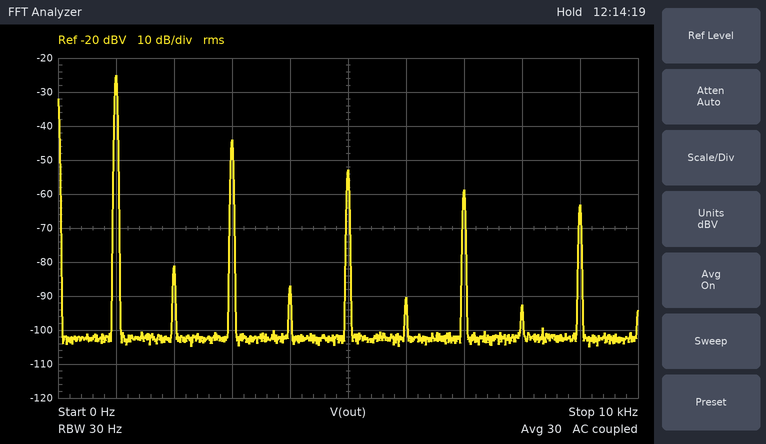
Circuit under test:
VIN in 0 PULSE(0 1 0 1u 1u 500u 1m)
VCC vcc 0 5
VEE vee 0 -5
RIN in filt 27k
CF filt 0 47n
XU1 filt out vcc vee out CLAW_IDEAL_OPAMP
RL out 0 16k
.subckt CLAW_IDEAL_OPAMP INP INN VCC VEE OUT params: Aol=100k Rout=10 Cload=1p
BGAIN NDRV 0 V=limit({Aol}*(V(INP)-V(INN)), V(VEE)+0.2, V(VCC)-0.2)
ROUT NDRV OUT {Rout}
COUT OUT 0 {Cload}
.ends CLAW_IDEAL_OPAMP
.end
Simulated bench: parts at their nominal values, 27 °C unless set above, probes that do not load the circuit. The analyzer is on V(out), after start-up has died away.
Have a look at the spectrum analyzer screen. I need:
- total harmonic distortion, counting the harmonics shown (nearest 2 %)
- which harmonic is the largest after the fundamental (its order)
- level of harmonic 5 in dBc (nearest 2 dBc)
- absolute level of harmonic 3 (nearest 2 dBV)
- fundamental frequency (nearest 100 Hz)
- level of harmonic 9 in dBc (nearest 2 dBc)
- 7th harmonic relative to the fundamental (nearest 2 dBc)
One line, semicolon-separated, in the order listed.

12 %; 3; -28 dBc; -44 dBV; 1.0 kHz; -38 dBc; -34 dBc
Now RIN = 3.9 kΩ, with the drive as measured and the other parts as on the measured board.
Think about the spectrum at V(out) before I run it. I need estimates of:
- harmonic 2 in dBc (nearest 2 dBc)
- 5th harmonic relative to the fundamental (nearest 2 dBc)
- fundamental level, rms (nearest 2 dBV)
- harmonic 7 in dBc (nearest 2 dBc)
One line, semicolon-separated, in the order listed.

-54 dBc; -26 dBc; -10 dBV; -32 dBc
